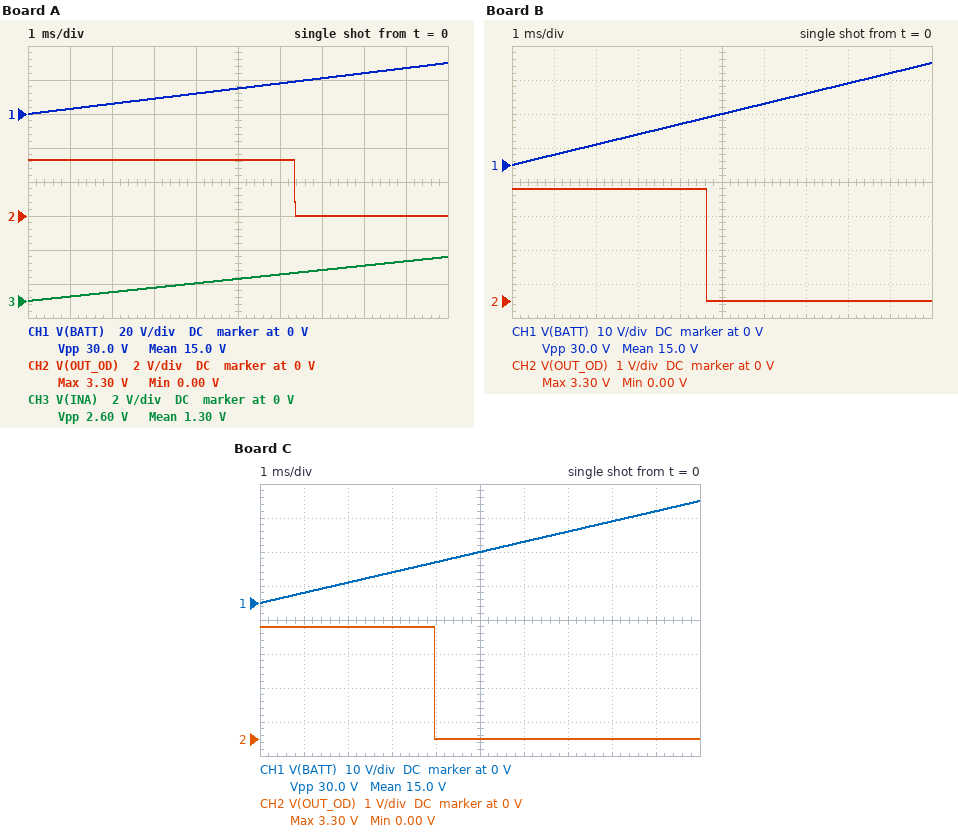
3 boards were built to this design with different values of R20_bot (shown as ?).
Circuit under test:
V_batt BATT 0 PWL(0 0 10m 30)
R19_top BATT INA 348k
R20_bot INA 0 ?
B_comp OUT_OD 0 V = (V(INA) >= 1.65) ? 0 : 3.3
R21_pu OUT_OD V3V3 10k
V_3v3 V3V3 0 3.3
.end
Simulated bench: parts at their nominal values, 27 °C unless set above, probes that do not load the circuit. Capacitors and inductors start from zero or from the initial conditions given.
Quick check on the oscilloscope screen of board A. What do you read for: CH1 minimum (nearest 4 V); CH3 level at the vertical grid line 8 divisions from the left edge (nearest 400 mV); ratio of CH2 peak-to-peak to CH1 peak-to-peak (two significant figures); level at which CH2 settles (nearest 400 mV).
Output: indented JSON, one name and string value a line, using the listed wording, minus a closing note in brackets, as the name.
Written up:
{
  "CH1 minimum": "0 V",
  "CH3 level at the vertical grid line 8 divisions from the left edge": "2.0 V",
  "ratio of CH2 peak-to-peak to CH1 peak-to-peak": "0.11",
  "level at which CH2 settles": "0 V"
}
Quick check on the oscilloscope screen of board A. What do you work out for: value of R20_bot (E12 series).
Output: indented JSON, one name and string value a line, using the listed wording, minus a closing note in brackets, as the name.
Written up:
{
  "value of R20_bot": "33 kΩ"
}
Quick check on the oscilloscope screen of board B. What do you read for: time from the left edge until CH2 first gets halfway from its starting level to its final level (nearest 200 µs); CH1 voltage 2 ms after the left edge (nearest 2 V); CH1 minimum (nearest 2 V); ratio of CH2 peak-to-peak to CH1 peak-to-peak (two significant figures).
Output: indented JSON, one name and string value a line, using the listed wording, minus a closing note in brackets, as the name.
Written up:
{
  "time from the left edge until CH2 first gets halfway from its starting level to its final level": "4.6 ms",
  "CH1 voltage 2 ms after the left edge": "6 V",
  "CH1 minimum": "0 V",
  "ratio of CH2 peak-to-peak to CH1 peak-to-peak": "0.11"
}
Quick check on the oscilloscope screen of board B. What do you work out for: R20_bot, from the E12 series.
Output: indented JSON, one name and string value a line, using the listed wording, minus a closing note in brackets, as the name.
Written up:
{
  "R20_bot, from the E12 series": "47 kΩ"
}
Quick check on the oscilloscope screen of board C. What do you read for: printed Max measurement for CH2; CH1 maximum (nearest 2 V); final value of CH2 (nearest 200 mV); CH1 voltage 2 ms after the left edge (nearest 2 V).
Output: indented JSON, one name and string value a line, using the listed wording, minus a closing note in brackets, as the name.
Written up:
{
  "printed Max measurement for CH2": "3.30 V",
  "CH1 maximum": "30 V",
  "final value of CH2": "0 V",
  "CH1 voltage 2 ms after the left edge": "6 V"
}
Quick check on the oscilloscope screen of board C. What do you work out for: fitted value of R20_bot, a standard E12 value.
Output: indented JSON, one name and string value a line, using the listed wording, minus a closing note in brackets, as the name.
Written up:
{
  "fitted value of R20_bot, a standard E12 value": "56 kΩ"
}
